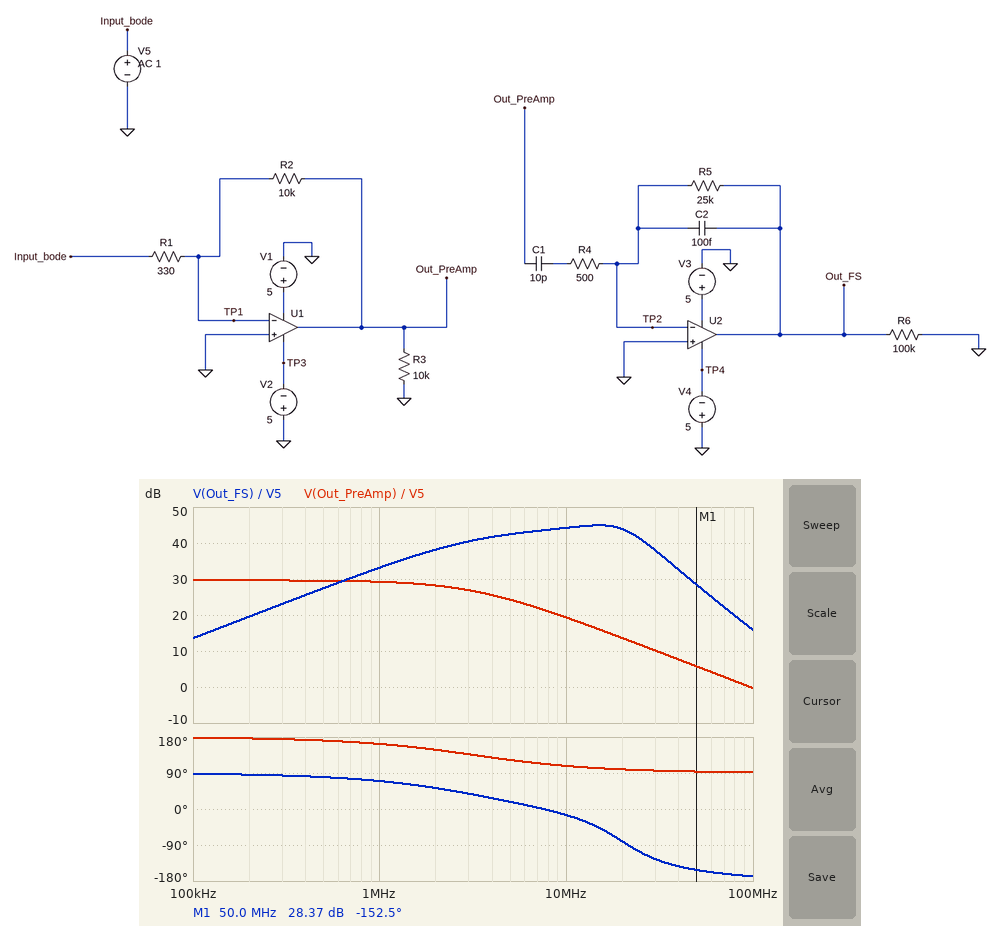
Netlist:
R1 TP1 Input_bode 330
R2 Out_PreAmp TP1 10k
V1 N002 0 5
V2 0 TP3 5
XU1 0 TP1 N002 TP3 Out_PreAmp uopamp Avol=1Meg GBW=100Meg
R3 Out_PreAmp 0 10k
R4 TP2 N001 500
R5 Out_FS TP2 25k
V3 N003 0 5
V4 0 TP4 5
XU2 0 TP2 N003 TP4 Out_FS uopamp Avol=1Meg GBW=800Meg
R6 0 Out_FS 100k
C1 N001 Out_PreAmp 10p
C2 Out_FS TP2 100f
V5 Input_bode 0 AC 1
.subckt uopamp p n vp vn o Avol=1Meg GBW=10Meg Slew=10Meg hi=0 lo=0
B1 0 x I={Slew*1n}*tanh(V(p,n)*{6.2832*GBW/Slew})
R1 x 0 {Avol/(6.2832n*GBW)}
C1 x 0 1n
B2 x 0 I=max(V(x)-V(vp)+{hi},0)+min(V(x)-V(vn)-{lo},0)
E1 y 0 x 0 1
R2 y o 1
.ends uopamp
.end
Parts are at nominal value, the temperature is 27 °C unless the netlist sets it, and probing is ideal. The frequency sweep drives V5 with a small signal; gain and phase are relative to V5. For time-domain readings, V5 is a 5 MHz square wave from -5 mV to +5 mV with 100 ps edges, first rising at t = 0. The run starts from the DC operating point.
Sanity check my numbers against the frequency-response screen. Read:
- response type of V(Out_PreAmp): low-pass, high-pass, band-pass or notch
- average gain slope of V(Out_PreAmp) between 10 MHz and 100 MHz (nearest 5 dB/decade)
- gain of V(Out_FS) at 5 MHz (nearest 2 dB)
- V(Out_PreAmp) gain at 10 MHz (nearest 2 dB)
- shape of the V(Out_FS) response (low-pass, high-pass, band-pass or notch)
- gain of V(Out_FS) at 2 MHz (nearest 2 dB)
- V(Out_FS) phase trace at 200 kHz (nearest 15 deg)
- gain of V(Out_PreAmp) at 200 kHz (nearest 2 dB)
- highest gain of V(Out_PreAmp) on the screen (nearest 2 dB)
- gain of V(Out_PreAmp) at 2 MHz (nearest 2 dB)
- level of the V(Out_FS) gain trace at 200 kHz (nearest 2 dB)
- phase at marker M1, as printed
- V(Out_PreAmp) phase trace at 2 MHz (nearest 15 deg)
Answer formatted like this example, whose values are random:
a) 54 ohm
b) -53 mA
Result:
a) low-pass
b) -20 dB/decade
c) 42 dB
d) 20 dB
e) band-pass
f) 38 dB
g) 90 deg
h) 30 dB
i) 30 dB
j) 28 dB
k) 20 dB
l) -152.5 deg
m) 150 deg
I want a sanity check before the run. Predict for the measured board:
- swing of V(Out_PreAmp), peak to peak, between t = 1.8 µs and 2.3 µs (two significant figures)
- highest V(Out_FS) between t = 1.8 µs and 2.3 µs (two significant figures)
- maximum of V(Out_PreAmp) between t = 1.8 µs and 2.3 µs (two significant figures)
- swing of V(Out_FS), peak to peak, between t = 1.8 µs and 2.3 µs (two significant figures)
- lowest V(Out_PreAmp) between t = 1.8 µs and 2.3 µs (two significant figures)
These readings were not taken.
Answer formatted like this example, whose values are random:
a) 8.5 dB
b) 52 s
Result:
a) 230 mV
b) 500 mV
c) 110 mV
d) 1.0 V
e) -110 mV
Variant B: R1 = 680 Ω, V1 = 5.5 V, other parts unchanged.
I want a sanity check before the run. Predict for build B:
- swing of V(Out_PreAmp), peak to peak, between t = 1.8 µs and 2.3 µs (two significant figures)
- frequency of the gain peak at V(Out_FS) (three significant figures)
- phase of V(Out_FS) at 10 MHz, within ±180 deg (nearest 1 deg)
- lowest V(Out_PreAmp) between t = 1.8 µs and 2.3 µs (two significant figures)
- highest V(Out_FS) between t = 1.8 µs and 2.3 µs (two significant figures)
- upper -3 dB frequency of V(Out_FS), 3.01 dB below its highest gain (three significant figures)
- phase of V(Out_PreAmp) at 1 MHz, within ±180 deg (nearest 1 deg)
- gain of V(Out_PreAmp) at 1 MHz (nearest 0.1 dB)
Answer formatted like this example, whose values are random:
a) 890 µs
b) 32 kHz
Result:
a) 140 mV
b) 15.7 MHz
c) 0 deg
d) -71 mV
e) 500 mV
f) 24.1 MHz
g) 171 deg
h) 23.2 dB
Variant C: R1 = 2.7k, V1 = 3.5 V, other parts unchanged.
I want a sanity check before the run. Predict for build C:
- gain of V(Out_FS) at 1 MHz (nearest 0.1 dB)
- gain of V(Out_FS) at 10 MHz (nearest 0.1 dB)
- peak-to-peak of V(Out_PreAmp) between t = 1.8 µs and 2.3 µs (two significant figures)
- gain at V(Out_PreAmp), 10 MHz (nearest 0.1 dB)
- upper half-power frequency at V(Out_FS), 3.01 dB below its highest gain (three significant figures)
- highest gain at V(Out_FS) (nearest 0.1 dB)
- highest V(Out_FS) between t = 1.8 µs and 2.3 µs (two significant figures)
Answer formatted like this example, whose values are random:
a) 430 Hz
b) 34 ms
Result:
a) 15.3 dB
b) 35.4 dB
c) 37 mV
d) 10.5 dB
e) 26.8 MHz
f) 39.1 dB
g) 330 mV
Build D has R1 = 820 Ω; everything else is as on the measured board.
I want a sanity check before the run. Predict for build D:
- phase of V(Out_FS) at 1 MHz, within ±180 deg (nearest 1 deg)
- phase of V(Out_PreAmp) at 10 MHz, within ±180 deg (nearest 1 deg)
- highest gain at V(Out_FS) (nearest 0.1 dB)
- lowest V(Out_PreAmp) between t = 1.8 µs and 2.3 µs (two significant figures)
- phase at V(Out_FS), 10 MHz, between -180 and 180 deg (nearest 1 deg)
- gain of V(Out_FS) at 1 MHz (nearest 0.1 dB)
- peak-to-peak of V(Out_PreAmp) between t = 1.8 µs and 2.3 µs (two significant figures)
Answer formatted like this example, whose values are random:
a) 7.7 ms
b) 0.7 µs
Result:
a) 80 deg
b) 127 deg
c) 43.8 dB
d) -60 mV
e) 4 deg
f) 25.6 dB
g) 120 mV
